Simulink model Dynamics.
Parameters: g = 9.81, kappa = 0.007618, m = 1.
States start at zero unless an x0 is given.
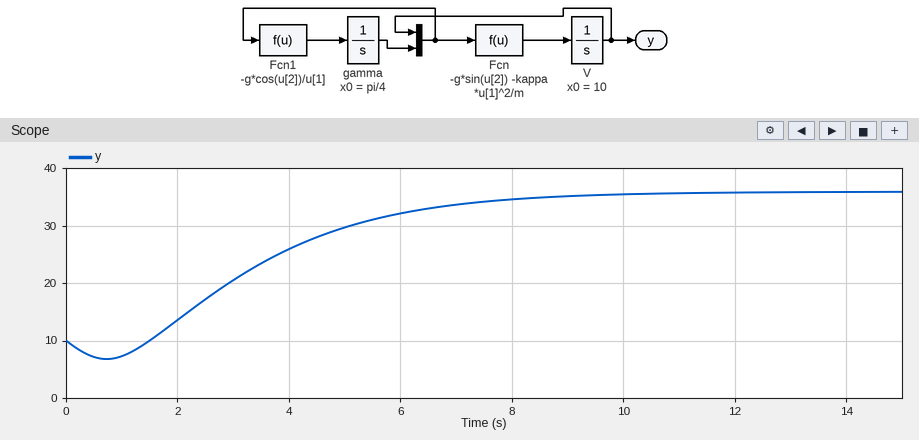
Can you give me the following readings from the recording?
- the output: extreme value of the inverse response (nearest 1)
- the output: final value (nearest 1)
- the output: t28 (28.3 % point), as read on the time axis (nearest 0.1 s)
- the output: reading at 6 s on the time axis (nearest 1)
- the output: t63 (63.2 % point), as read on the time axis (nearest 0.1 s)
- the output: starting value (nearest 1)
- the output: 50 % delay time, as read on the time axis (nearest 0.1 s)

7
36
2.5 s
32
4.1 s
10
3.4 s
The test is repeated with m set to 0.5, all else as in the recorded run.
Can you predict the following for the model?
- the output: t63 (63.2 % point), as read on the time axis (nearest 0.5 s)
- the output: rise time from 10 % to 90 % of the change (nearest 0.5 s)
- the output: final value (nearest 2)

3.5 s
3.5 s
26
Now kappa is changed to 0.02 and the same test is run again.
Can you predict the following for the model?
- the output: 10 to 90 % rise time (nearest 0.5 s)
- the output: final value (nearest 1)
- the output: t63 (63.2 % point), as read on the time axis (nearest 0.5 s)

3.0 s
22
3.0 s
